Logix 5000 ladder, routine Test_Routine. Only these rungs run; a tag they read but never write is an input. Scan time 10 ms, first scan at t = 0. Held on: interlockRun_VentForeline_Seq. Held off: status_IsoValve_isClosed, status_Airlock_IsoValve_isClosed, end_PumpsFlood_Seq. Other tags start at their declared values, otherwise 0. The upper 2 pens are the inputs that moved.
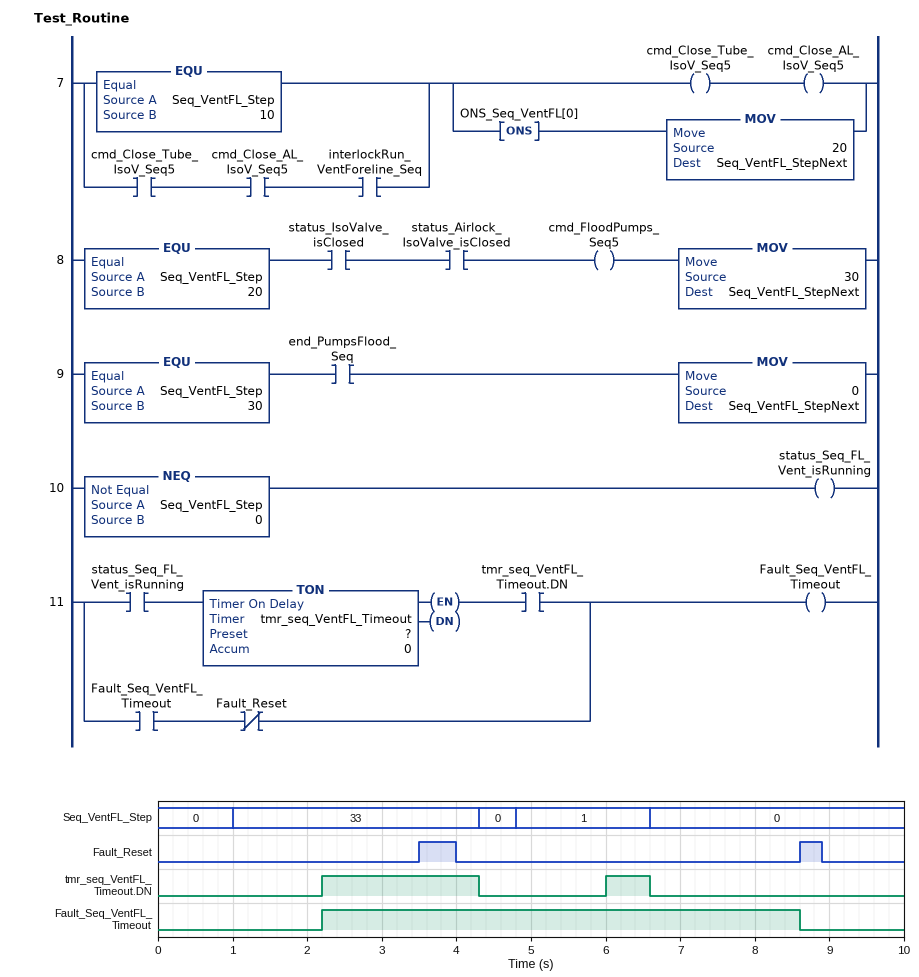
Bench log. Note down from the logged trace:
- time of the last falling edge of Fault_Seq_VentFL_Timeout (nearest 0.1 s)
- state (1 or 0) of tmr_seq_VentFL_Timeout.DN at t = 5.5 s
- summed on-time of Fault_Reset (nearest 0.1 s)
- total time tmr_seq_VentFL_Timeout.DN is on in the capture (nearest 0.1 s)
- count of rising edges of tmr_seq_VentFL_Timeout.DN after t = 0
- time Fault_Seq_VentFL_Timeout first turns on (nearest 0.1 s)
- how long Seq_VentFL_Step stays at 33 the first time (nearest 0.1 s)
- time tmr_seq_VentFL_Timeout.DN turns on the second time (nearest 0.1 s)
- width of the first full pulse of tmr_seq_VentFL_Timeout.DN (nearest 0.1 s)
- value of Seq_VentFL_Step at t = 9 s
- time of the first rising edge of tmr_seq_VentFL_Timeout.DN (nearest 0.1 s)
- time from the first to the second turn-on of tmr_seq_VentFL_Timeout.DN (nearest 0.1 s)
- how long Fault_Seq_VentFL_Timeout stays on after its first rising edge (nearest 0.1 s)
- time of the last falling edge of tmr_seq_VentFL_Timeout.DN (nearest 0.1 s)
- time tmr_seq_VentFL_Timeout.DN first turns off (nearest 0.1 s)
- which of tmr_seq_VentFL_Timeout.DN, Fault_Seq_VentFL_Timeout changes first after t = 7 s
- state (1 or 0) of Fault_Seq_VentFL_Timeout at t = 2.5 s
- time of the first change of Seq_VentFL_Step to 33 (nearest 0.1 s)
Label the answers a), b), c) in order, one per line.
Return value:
a) 8.6 s
b) 0
c) 0.8 s
d) 2.7 s
e) 2
f) 2.2 s
g) 3.3 s
h) 6.0 s
i) 2.1 s
j) 0
k) 2.2 s
l) 3.8 s
m) 6.4 s
n) 6.6 s
o) 4.3 s
p) Fault_Seq_VentFL_Timeout
q) 1
r) 1.0 s
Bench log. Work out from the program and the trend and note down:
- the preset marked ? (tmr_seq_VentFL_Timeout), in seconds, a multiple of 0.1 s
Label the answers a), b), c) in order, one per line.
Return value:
a) 1.2 s
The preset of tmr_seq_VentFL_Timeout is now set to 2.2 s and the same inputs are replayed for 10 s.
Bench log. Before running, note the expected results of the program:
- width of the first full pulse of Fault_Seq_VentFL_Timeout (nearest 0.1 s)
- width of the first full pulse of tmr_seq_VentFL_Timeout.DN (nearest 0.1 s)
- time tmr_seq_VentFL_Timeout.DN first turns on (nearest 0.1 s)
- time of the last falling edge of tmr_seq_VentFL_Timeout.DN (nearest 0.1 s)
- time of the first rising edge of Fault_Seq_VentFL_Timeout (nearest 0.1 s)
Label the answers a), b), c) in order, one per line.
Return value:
a) 5.4 s
b) 1.1 s
c) 3.2 s
d) 4.3 s
e) 3.2 s
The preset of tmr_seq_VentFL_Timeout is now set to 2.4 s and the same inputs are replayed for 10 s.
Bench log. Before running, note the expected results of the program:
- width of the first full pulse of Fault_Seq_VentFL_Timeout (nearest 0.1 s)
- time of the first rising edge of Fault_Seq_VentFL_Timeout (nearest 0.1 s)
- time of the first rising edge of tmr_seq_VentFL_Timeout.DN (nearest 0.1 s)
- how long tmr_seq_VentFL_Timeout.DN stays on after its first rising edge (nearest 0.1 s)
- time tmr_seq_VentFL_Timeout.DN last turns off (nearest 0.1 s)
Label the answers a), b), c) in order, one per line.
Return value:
a) 5.2 s
b) 3.4 s
c) 3.4 s
d) 0.9 s
e) 4.3 s
